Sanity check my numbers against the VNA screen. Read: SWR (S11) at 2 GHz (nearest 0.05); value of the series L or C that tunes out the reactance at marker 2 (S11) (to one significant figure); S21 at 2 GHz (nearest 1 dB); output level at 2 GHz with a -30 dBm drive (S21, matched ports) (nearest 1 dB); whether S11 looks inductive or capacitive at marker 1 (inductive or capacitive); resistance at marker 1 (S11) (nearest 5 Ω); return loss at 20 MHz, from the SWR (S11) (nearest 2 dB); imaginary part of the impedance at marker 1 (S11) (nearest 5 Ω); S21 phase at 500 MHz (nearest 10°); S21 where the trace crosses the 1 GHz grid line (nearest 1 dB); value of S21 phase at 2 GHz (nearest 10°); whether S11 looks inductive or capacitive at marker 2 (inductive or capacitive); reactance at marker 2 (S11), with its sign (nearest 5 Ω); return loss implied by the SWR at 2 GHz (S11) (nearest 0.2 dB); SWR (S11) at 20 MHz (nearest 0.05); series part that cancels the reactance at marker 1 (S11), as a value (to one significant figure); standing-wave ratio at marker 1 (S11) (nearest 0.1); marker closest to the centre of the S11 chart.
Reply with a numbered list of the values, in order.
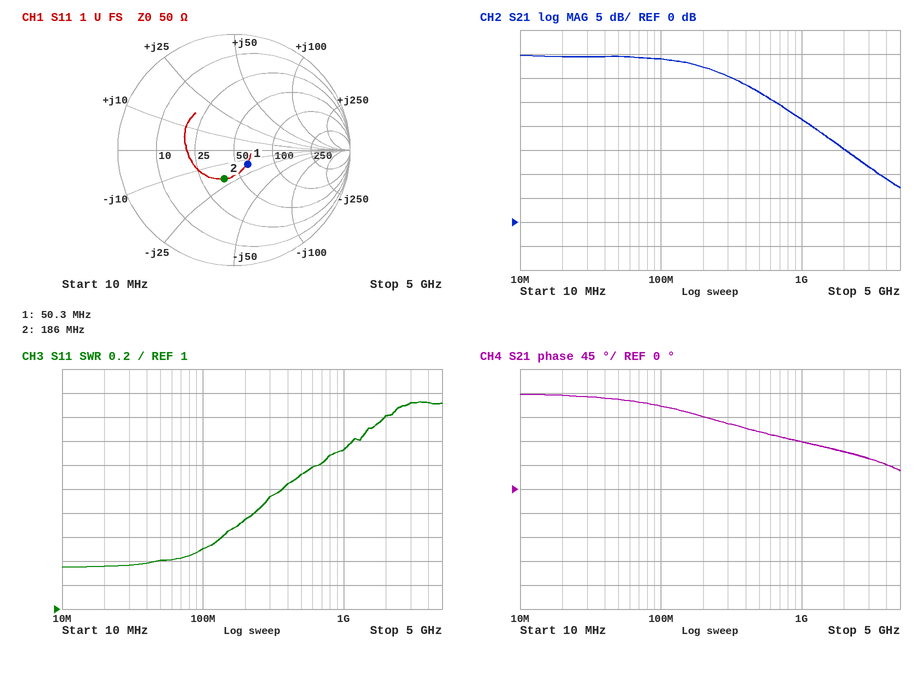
1. 2.60
2. 20 nH
3. 15 dB
4. -15 dBm
5. capacitive
6. 60 Ω
7. 16 dB
8. -15 Ω
9. 110°
10. 21 dB
11. 70°
12. capacitive
13. -20 Ω
14. 7.0 dB
15. 1.35
16. 50 nH
17. 1.4
18. marker 1
